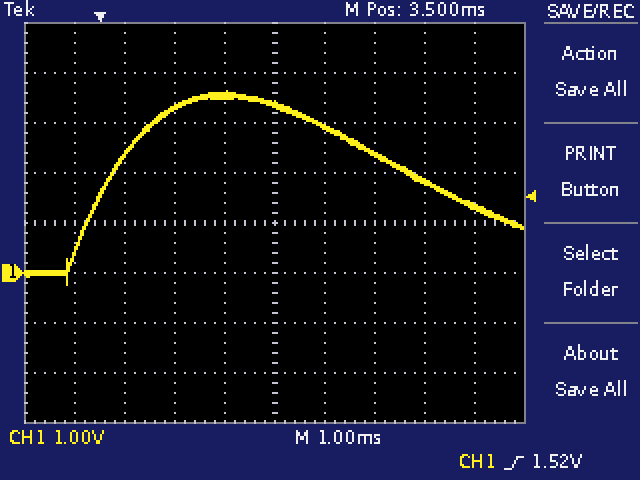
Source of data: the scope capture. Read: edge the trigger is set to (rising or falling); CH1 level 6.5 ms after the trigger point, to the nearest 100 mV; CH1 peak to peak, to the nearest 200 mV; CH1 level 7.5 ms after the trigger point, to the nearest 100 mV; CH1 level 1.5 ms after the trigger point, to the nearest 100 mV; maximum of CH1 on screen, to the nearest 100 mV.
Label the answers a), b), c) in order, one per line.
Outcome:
a) rising
b) 1.8 V
c) 3.8 V
d) 1.3 V
e) 3.3 V
f) 3.6 V
